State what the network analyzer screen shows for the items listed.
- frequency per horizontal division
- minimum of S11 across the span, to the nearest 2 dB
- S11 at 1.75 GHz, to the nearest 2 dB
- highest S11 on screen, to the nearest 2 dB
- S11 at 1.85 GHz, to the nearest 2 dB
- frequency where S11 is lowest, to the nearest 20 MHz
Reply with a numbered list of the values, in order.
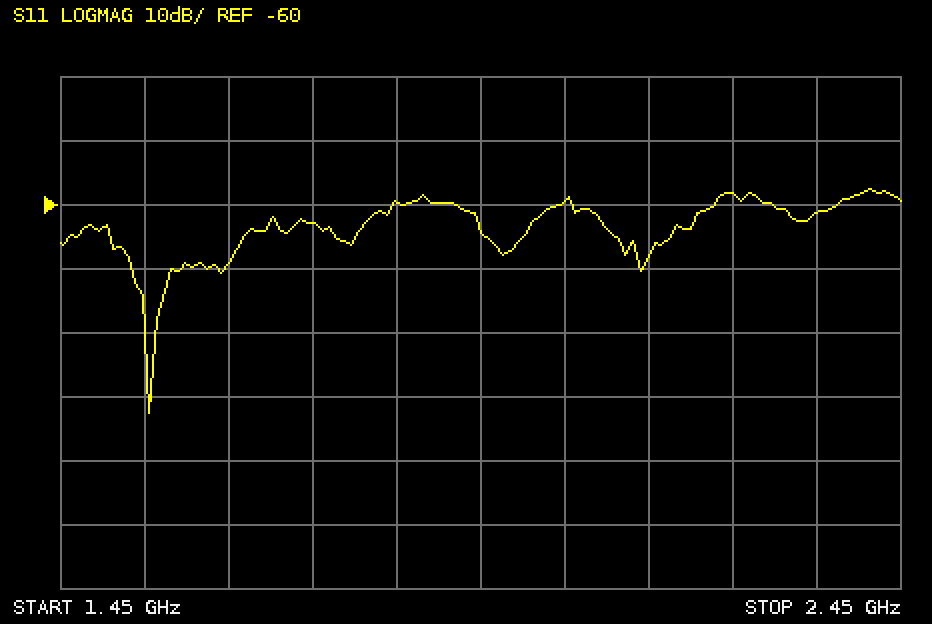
1. 100 MHz
2. -92 dB
3. -62 dB
4. -58 dB
5. -60 dB
6. 1.56 GHz
